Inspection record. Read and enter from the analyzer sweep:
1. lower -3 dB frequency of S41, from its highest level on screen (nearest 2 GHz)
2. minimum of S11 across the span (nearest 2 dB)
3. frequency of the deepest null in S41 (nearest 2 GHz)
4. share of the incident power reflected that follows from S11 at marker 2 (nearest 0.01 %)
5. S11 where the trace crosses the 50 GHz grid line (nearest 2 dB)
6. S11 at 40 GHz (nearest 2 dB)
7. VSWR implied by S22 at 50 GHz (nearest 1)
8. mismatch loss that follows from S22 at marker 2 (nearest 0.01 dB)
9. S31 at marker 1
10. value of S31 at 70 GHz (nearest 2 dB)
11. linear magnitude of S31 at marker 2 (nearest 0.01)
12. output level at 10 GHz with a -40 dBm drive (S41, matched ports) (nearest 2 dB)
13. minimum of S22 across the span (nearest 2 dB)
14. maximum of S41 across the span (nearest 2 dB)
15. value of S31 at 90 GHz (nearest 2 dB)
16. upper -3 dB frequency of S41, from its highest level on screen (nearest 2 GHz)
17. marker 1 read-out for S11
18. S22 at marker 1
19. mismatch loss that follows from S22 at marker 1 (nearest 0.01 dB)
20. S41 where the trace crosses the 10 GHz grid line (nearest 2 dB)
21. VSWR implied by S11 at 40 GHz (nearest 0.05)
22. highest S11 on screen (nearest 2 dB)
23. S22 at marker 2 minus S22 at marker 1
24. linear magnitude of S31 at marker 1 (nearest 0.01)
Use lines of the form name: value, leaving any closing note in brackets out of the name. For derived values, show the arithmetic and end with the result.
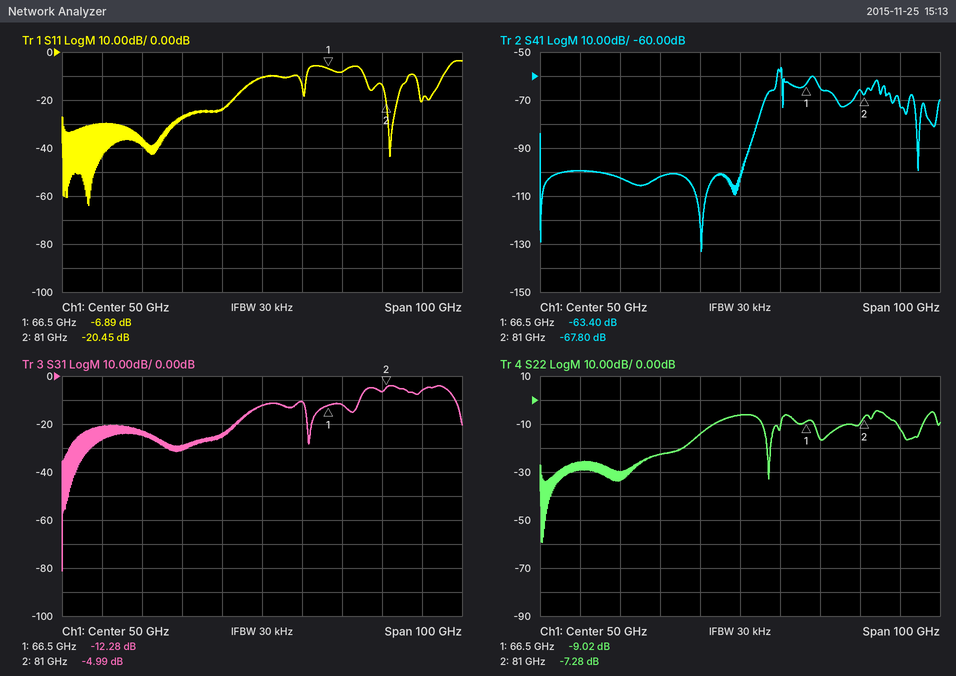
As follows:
lower -3 dB frequency of S41, from its highest level on screen: 60 GHz
minimum of S11 across the span: -64 dB
frequency of the deepest null in S41: 40 GHz
share of the incident power reflected that follows from S11 at marker 2: 10^(-20.45/10) ≈ 0.90 %
S11 where the trace crosses the 50 GHz grid line: -10 dB
S11 at 40 GHz: -24 dB
VSWR implied by S22 at 50 GHz: |Γ| = 10^(-6/20) = 0.5012; VSWR = (1 + 0.5012)/(1 − 0.5012) ≈ 3
mismatch loss that follows from S22 at marker 2: −10 log10(1 − 10^(-7.28/10)) ≈ 0.90 dB
S31 at marker 1: -12.28 dB
value of S31 at 70 GHz: -12 dB
linear magnitude of S31 at marker 2: 10^(-4.99/20) ≈ 0.56
output level at 10 GHz with a -40 dBm drive (S41, matched ports): -40 dBm + (-100 dB) = -140 dBm
minimum of S22 across the span: -60 dB
maximum of S41 across the span: -56 dB
value of S31 at 90 GHz: -6 dB
upper -3 dB frequency of S41, from its highest level on screen: 60 GHz
marker 1 read-out for S11: -6.89 dB
S22 at marker 1: -9.02 dB
mismatch loss that follows from S22 at marker 1: −10 log10(1 − 10^(-9.02/10)) ≈ 0.58 dB
S41 where the trace crosses the 10 GHz grid line: -100 dB
VSWR implied by S11 at 40 GHz: |Γ| = 10^(-24/20) = 0.0631; VSWR = (1 + 0.0631)/(1 − 0.0631) ≈ 1.13, so 1.15 to the nearest 0.05
highest S11 on screen: -4 dB
S22 at marker 2 minus S22 at marker 1: -7.28 − (-9.02) = 1.74 dB
linear magnitude of S31 at marker 1: 10^(-12.28/20) ≈ 0.24
